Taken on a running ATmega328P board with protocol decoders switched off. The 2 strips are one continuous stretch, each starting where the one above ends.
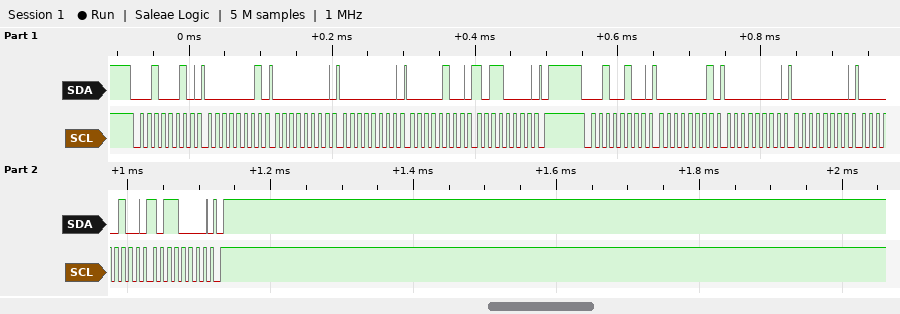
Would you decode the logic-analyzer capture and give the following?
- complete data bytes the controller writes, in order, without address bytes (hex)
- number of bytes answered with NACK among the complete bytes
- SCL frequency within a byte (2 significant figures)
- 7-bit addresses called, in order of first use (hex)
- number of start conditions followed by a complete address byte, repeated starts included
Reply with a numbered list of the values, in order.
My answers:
1. 01 00 00 04 B0 01 00 00 04 B0
2. 0
3. 100 kHz
4. 0x11 0x12
5. 2
